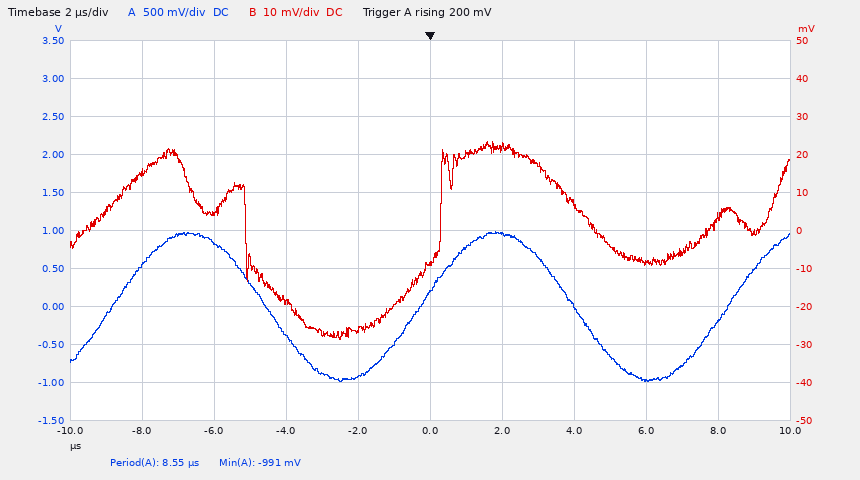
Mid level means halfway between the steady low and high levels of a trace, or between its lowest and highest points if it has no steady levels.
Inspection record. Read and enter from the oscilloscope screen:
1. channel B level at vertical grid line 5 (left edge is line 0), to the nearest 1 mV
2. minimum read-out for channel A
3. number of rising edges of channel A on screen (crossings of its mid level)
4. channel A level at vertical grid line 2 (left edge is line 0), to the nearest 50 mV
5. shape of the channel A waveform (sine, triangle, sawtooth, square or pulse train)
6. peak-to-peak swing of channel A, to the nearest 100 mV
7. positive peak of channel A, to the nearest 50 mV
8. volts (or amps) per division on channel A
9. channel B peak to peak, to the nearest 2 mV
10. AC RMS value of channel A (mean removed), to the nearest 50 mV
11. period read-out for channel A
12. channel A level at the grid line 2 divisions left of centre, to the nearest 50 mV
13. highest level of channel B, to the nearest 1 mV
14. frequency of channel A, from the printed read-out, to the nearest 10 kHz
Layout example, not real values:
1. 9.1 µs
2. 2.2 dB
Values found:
1. -9 mV
2. -991 mV
3. 3
4. 850 mV
5. sine
6. 2.00 V
7. 1.00 V
8. 500 mV
9. 52 mV
10. 700 mV
11. 8.55 µs
12. -400 mV
13. 23 mV
14. 120 kHz
